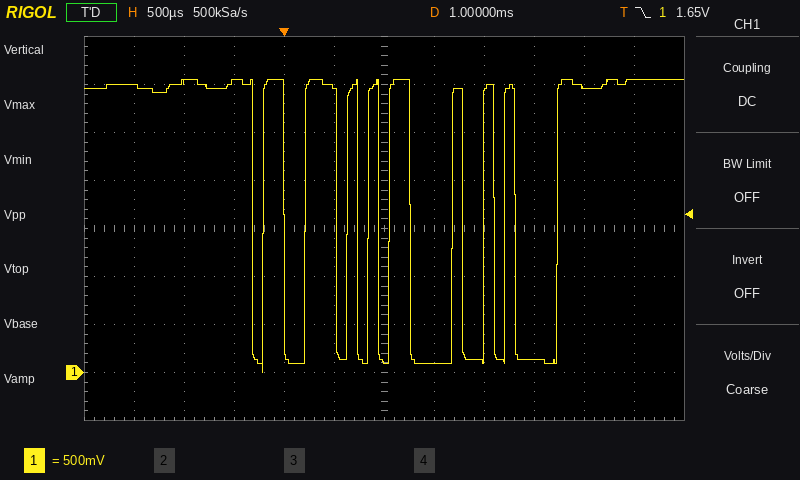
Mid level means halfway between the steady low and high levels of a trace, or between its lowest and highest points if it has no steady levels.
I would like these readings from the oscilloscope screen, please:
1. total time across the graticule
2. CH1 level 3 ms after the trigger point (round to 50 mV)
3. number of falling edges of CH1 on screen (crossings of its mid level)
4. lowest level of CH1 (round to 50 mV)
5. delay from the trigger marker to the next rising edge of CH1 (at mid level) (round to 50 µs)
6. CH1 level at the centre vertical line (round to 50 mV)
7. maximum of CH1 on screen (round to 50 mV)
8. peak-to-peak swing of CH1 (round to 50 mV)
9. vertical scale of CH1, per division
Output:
6 ms
3.00 V
9
0 mV
200 µs
100 mV
3.05 V
3.05 V
500 mV
